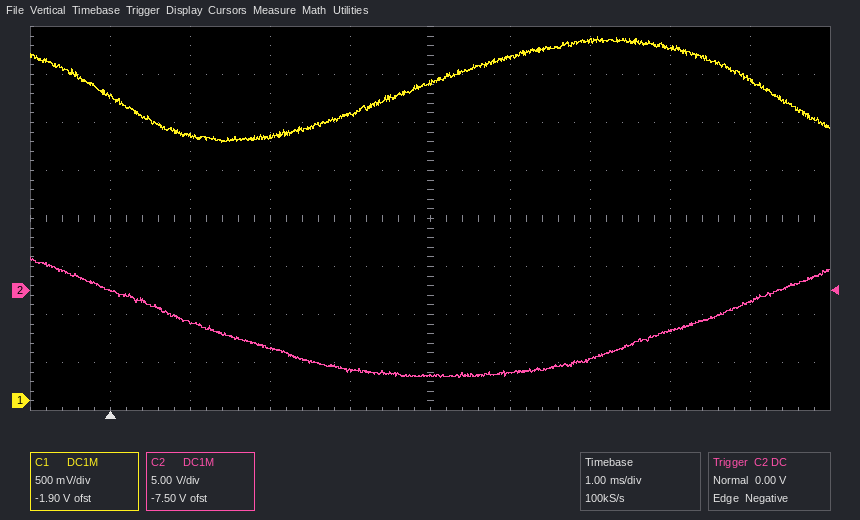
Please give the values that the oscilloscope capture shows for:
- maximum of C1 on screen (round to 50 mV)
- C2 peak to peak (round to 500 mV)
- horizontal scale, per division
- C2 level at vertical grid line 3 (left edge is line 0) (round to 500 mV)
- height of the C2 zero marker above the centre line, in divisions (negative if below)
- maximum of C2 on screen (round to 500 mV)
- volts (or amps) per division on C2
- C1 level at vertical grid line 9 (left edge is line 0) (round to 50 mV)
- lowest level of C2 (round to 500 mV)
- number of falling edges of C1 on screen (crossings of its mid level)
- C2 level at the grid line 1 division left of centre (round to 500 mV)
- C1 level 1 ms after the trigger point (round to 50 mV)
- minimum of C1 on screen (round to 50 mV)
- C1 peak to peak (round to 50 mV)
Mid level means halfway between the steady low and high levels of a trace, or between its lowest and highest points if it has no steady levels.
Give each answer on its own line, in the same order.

3.80 V
12.5 V
1 ms
-6.0 V
-1.5 div
3.5 V
5 V
3.35 V
-9.0 V
2
-8.5 V
2.75 V
2.70 V
1.10 V
